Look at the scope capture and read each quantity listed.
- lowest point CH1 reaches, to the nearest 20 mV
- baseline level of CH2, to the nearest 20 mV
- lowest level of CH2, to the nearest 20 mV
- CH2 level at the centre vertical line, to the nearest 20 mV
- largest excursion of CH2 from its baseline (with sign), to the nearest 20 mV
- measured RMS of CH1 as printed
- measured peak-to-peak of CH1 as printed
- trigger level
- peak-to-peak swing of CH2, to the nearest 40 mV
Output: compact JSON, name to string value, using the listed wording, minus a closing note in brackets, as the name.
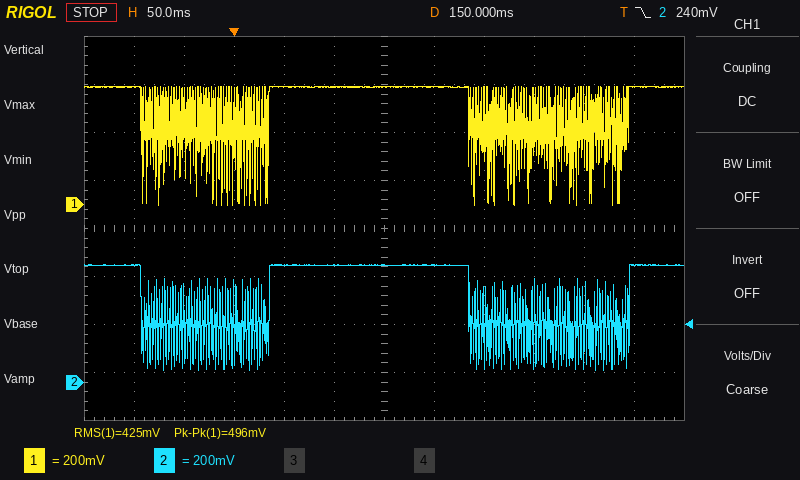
{"lowest point CH1 reaches, to the nearest 20 mV": "0 mV", "baseline level of CH2, to the nearest 20 mV": "480 mV", "lowest level of CH2, to the nearest 20 mV": "40 mV", "CH2 level at the centre vertical line, to the nearest 20 mV": "480 mV", "largest excursion of CH2 from its baseline (with sign), to the nearest 20 mV": "-440 mV", "measured RMS of CH1 as printed": "425 mV", "measured peak-to-peak of CH1 as printed": "496 mV", "trigger level": "240 mV", "peak-to-peak swing of CH2, to the nearest 40 mV": "440 mV"}
